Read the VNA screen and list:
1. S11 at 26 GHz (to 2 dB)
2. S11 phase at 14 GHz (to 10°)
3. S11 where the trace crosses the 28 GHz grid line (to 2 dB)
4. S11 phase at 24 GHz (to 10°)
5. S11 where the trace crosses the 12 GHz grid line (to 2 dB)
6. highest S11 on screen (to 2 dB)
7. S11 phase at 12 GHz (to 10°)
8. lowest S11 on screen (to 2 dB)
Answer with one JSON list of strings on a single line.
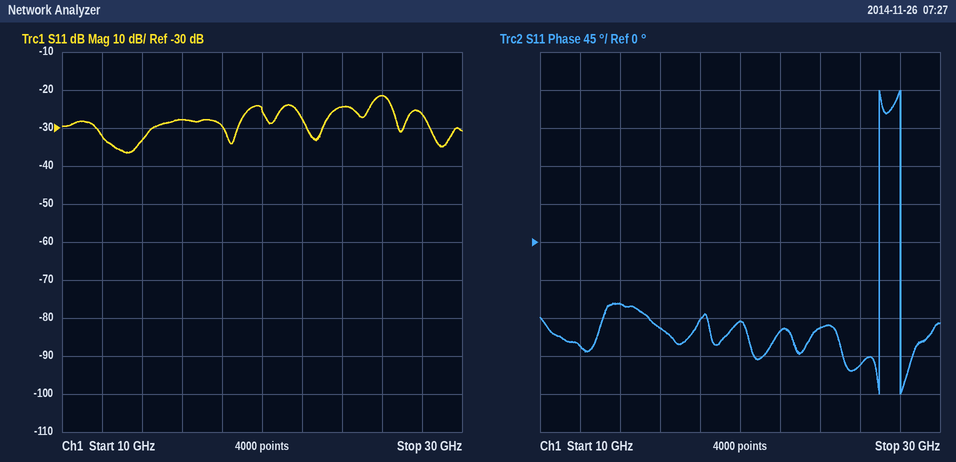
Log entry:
["-22 dB", "-70°", "-26 dB", "-100°", "-32 dB", "-22 dB", "-120°", "-36 dB"]
